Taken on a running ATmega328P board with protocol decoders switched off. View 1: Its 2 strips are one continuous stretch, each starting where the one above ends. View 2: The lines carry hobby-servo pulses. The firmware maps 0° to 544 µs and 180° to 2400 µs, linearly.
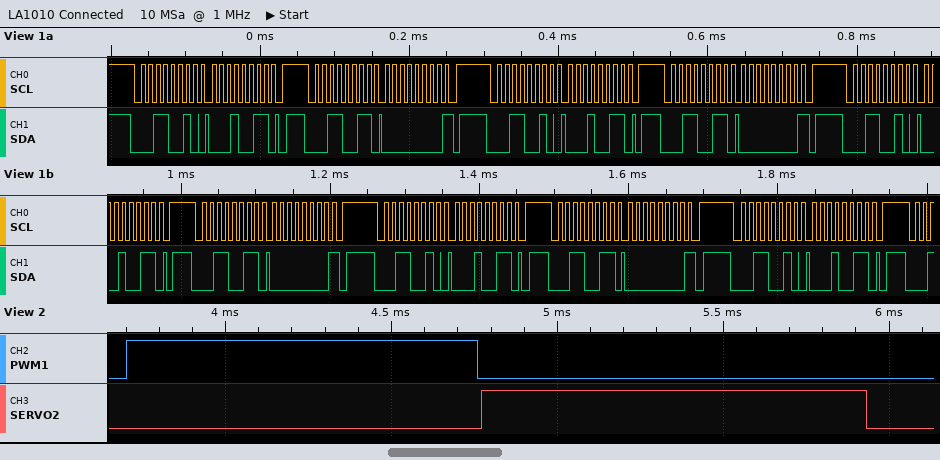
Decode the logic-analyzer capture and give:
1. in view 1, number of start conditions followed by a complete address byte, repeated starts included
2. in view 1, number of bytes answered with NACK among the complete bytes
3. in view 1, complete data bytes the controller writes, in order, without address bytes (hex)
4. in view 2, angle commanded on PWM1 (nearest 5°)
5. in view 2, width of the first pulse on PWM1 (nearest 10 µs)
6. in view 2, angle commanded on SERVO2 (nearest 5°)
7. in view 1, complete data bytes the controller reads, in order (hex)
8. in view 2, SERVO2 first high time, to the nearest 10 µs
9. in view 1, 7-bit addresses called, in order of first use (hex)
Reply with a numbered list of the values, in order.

1. 9
2. 4
3. 13 13 13 13 13
4. 50°
5. 1060 µs
6. 60°
7. 00 00 00 00
8. 1160 µs
9. 0x19
